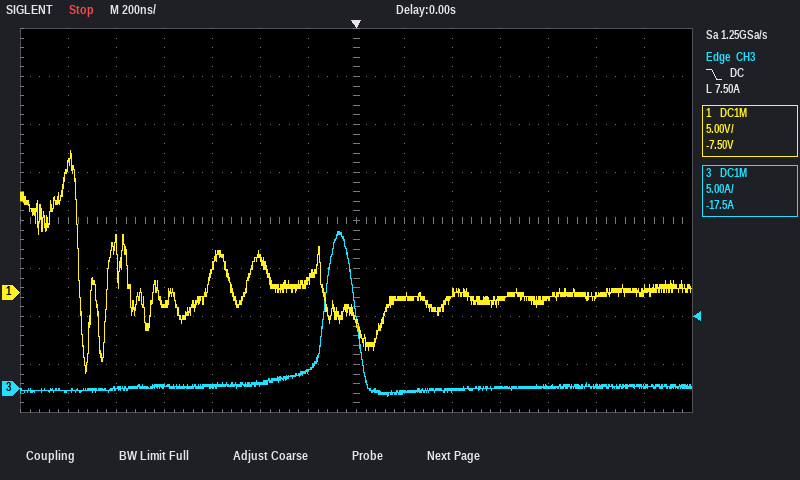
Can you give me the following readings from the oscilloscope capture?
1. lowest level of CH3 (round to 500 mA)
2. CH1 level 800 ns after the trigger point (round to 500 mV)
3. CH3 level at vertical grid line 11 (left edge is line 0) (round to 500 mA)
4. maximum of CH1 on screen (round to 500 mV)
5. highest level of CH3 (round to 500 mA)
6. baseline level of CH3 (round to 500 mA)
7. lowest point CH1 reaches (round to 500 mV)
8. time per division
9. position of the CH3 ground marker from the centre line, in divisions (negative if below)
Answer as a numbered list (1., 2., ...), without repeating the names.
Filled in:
1. -1.0 A
2. -500 mV
3. 0.0 A
4. 15.0 V
5. 16.5 A
6. 0.0 A
7. -8.5 V
8. 200 ns
9. -3.5 div
